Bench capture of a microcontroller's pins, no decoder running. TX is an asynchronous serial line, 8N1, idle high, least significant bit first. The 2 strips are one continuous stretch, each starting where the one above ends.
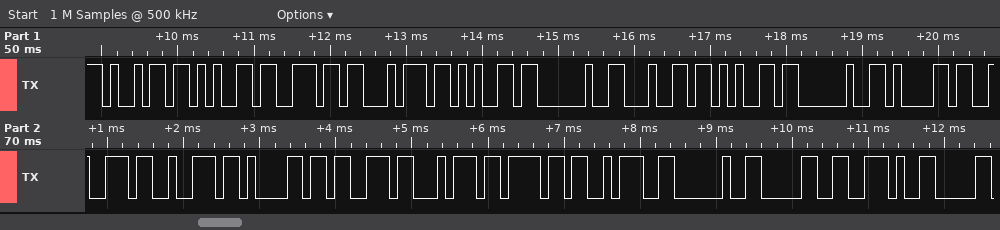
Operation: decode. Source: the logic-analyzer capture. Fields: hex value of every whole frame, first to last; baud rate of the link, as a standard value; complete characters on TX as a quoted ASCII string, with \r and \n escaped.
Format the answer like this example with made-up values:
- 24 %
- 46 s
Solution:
- 0x69 0x65 0x6E 0x74 0x65 0x20 0x64 0x65 0x20 0x61 0x72 0x72 0x61 0x73 0x74 0x6F 0x3A 0x20 0x30 0x2E
- 9600 baud
- "iente de arrasto: 0."
